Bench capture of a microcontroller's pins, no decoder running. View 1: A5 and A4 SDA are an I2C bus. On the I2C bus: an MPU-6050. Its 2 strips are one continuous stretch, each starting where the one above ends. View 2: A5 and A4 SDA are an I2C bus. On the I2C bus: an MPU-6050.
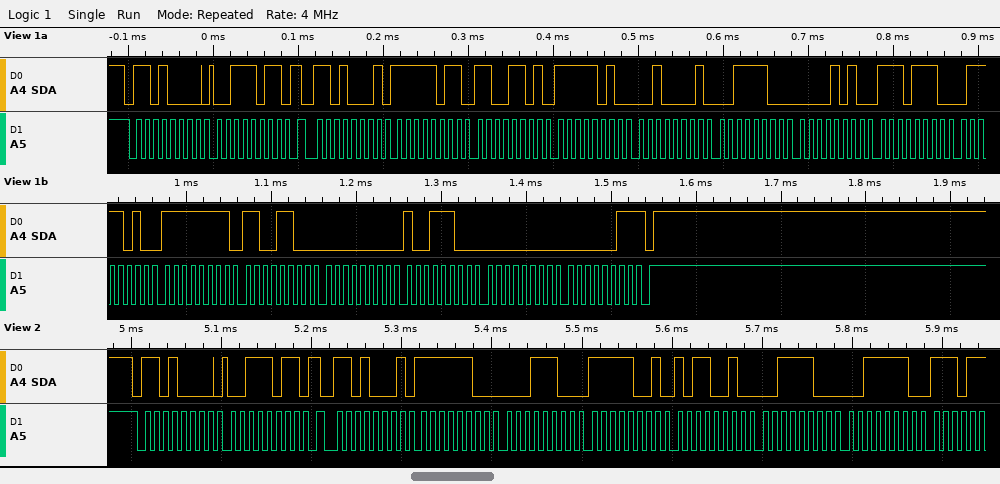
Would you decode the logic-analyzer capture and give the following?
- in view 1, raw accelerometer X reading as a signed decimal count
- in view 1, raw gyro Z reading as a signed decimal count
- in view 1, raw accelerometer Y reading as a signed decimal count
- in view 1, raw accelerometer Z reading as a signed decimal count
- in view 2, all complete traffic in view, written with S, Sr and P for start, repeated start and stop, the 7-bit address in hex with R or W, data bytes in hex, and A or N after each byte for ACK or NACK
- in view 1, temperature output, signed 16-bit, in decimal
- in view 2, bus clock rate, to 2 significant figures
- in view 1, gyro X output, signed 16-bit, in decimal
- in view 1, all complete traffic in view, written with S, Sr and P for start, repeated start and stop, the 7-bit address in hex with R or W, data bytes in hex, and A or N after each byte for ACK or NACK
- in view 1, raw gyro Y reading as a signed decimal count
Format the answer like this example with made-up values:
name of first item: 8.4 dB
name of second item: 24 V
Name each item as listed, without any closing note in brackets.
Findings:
in view 1, raw accelerometer X reading as a signed decimal count: -1075
in view 1, raw gyro Z reading as a signed decimal count: 3
in view 1, raw accelerometer Y reading as a signed decimal count: -1503
in view 1, raw accelerometer Z reading as a signed decimal count: 15370
in view 2, all complete traffic in view, written with S, Sr and P for start, repeated start and stop, the 7-bit address in hex with R or W, data bytes in hex, and A or N after each byte for ACK or NACK: S 68W A 3B A Sr 68R A FC A 1C A F9 A B2 A 3C A 3E A
in view 1, temperature output, signed 16-bit, in decimal: -4486
in view 2, bus clock rate, to 2 significant figures: 100 kHz
in view 1, gyro X output, signed 16-bit, in decimal: -52
in view 1, all complete traffic in view, written with S, Sr and P for start, repeated start and stop, the 7-bit address in hex with R or W, data bytes in hex, and A or N after each byte for ACK or NACK: S 68W A 3B A Sr 68R A FB A CD A FA A 21 A 3C A 0A A EE A 7A A FF A CC A 00 A 9C A 00 A 03 N P
in view 1, raw gyro Y reading as a signed decimal count: 156
